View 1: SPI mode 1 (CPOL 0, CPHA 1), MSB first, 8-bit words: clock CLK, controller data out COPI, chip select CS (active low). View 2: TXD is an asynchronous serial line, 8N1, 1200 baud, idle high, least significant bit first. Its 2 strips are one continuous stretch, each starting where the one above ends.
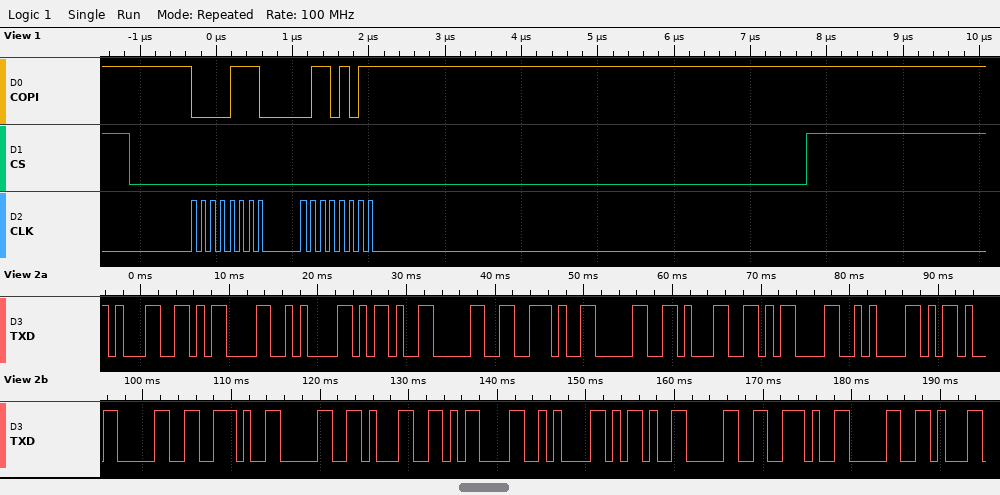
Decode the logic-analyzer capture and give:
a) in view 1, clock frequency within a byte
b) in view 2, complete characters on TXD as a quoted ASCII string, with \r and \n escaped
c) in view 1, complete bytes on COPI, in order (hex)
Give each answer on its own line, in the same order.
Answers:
8 MHz
"1\r\n-0.01\r\n-0.01\r\n-0.0"
0E 6B
